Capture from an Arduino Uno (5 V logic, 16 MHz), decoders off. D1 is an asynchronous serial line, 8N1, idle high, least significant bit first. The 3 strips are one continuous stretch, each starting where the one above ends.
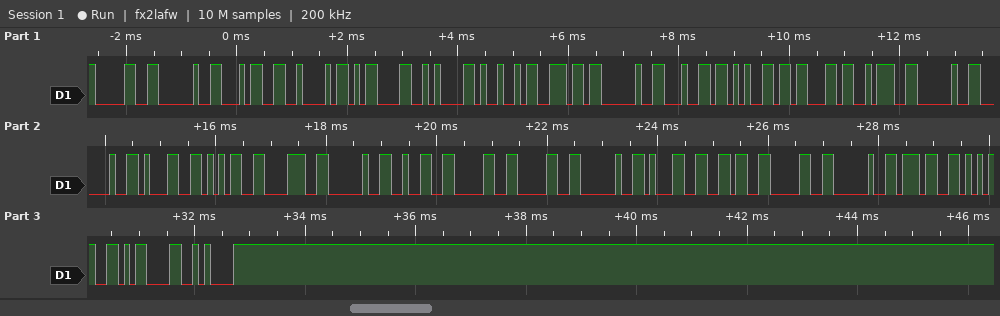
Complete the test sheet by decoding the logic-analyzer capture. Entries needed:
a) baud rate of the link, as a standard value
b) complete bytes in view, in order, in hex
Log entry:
9600 baud
30 20 34 42 0D 0A 49 6E 20 64 65 63 3A 20 20 31 35 38 20 32 30 30 20 31 36 30 20 37 35 0D 0A
